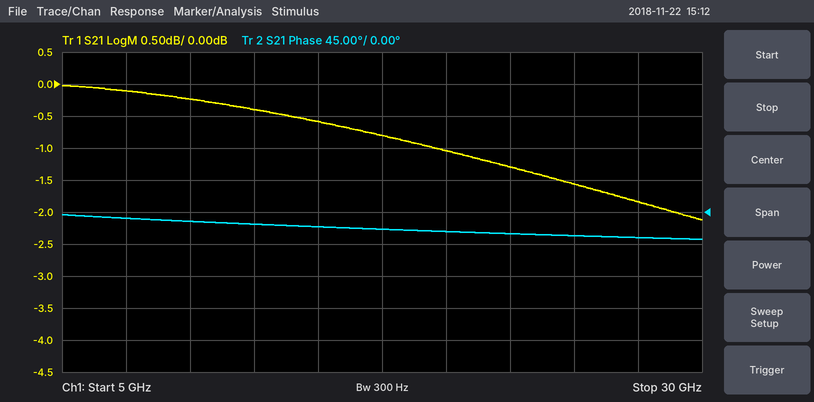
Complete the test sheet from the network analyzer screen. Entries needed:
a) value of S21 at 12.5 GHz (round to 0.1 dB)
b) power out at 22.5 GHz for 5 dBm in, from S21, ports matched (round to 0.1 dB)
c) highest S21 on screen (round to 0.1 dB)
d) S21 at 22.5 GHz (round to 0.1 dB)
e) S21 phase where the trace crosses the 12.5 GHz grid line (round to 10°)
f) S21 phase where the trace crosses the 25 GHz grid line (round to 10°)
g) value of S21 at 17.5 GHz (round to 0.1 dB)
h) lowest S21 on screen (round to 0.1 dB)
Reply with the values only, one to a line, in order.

-0.4 dB
3.7 dBm
0.0 dB
-1.3 dB
-20°
-30°
-0.8 dB
-2.1 dB
